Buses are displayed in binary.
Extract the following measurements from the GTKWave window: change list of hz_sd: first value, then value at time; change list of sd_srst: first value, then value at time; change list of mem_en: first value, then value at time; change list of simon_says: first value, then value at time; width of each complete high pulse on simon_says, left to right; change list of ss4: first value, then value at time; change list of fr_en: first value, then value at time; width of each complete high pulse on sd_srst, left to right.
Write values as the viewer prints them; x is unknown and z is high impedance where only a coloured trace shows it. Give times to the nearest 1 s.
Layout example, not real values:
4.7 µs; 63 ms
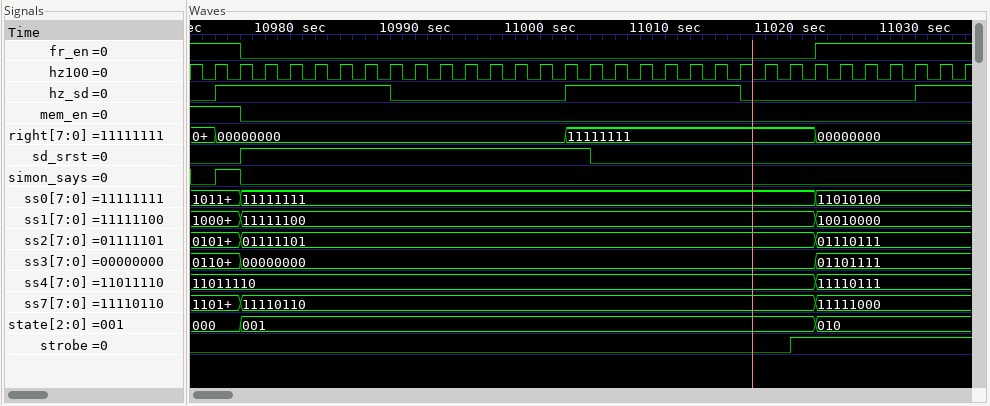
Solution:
0, 1 at 10974 s, 0 at 10988 s, 1 at 11002 s, 0 at 11016 s, 1 at 11030 s; 0, 1 at 10976 s, 0 at 11004 s; 1, 0 at 10976 s; 0, 1 at 10974 s, 0 at 10976 s; 2 s; 11011110, 11110111 at 11022 s; 1, 0 at 10976 s, 1 at 11022 s; 28 s
